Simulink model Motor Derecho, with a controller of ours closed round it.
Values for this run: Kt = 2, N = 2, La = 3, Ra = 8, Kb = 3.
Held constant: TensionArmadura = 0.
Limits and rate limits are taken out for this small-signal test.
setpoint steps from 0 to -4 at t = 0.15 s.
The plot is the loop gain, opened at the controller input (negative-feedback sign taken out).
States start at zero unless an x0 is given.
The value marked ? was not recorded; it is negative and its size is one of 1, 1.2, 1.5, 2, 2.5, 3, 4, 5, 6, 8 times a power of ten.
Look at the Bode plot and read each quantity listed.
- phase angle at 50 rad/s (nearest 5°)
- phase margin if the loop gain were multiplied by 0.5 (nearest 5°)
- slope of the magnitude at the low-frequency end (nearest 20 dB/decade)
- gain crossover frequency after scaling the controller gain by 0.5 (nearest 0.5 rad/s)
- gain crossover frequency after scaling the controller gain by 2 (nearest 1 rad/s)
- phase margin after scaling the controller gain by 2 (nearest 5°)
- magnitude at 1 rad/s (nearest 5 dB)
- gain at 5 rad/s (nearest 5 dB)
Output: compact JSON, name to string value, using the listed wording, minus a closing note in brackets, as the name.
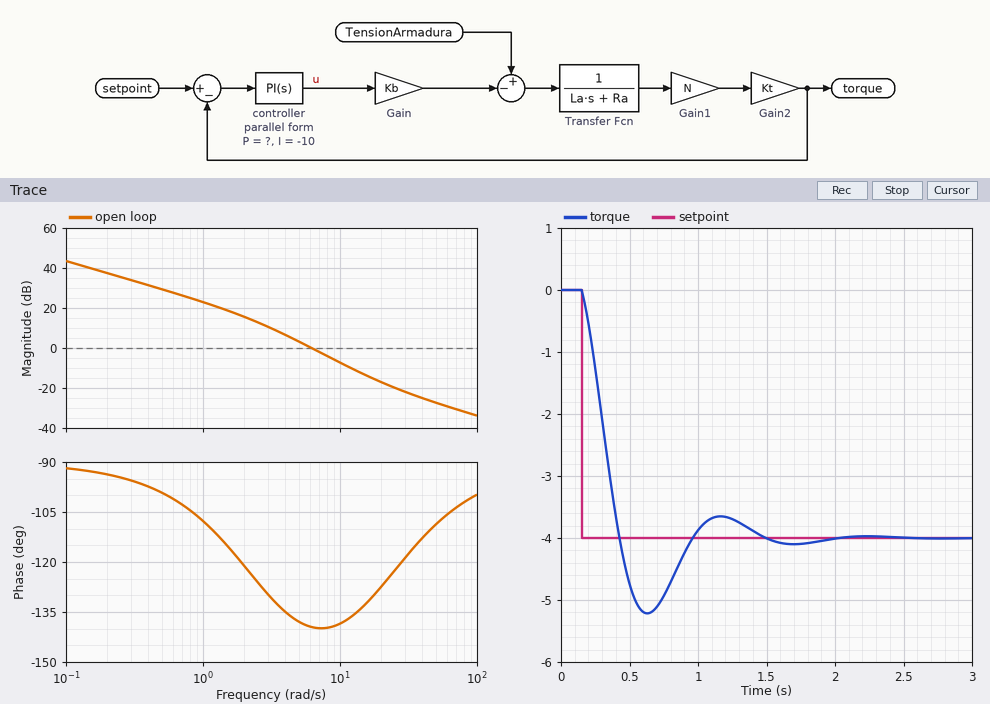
{"phase angle at 50 rad/s": "-110°", "phase margin if the loop gain were multiplied by 0.5": "45°", "slope of the magnitude at the low-frequency end": "-20 dB/decade", "gain crossover frequency after scaling the controller gain by 0.5": "4.0 rad/s", "gain crossover frequency after scaling the controller gain by 2": "9 rad/s", "phase margin after scaling the controller gain by 2": "40°", "magnitude at 1 rad/s": "25 dB", "gain at 5 rad/s": "5 dB"}
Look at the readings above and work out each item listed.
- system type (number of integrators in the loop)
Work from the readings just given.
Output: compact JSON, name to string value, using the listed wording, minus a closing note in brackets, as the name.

{"system type": "1"}
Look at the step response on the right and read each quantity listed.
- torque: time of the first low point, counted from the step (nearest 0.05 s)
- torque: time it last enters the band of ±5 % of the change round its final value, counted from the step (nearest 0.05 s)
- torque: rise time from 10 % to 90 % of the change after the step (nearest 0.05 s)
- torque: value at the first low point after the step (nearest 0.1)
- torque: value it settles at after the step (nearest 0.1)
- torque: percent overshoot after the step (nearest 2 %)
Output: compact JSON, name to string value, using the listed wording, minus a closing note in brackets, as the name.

{"torque: time of the first low point, counted from the step": "0.50 s", "torque: time it last enters the band of ±5 % of the change round its final value, counted from the step": "1.20 s", "torque: rise time from 10 % to 90 % of the change after the step": "0.20 s", "torque: value at the first low point after the step": "-5.2", "torque: value it settles at after the step": "-4.0", "torque: percent overshoot after the step": "30 %"}
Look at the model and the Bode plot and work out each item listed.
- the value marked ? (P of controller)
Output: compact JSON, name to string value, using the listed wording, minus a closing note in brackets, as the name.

{"the value marked ?": "-0.5"}
